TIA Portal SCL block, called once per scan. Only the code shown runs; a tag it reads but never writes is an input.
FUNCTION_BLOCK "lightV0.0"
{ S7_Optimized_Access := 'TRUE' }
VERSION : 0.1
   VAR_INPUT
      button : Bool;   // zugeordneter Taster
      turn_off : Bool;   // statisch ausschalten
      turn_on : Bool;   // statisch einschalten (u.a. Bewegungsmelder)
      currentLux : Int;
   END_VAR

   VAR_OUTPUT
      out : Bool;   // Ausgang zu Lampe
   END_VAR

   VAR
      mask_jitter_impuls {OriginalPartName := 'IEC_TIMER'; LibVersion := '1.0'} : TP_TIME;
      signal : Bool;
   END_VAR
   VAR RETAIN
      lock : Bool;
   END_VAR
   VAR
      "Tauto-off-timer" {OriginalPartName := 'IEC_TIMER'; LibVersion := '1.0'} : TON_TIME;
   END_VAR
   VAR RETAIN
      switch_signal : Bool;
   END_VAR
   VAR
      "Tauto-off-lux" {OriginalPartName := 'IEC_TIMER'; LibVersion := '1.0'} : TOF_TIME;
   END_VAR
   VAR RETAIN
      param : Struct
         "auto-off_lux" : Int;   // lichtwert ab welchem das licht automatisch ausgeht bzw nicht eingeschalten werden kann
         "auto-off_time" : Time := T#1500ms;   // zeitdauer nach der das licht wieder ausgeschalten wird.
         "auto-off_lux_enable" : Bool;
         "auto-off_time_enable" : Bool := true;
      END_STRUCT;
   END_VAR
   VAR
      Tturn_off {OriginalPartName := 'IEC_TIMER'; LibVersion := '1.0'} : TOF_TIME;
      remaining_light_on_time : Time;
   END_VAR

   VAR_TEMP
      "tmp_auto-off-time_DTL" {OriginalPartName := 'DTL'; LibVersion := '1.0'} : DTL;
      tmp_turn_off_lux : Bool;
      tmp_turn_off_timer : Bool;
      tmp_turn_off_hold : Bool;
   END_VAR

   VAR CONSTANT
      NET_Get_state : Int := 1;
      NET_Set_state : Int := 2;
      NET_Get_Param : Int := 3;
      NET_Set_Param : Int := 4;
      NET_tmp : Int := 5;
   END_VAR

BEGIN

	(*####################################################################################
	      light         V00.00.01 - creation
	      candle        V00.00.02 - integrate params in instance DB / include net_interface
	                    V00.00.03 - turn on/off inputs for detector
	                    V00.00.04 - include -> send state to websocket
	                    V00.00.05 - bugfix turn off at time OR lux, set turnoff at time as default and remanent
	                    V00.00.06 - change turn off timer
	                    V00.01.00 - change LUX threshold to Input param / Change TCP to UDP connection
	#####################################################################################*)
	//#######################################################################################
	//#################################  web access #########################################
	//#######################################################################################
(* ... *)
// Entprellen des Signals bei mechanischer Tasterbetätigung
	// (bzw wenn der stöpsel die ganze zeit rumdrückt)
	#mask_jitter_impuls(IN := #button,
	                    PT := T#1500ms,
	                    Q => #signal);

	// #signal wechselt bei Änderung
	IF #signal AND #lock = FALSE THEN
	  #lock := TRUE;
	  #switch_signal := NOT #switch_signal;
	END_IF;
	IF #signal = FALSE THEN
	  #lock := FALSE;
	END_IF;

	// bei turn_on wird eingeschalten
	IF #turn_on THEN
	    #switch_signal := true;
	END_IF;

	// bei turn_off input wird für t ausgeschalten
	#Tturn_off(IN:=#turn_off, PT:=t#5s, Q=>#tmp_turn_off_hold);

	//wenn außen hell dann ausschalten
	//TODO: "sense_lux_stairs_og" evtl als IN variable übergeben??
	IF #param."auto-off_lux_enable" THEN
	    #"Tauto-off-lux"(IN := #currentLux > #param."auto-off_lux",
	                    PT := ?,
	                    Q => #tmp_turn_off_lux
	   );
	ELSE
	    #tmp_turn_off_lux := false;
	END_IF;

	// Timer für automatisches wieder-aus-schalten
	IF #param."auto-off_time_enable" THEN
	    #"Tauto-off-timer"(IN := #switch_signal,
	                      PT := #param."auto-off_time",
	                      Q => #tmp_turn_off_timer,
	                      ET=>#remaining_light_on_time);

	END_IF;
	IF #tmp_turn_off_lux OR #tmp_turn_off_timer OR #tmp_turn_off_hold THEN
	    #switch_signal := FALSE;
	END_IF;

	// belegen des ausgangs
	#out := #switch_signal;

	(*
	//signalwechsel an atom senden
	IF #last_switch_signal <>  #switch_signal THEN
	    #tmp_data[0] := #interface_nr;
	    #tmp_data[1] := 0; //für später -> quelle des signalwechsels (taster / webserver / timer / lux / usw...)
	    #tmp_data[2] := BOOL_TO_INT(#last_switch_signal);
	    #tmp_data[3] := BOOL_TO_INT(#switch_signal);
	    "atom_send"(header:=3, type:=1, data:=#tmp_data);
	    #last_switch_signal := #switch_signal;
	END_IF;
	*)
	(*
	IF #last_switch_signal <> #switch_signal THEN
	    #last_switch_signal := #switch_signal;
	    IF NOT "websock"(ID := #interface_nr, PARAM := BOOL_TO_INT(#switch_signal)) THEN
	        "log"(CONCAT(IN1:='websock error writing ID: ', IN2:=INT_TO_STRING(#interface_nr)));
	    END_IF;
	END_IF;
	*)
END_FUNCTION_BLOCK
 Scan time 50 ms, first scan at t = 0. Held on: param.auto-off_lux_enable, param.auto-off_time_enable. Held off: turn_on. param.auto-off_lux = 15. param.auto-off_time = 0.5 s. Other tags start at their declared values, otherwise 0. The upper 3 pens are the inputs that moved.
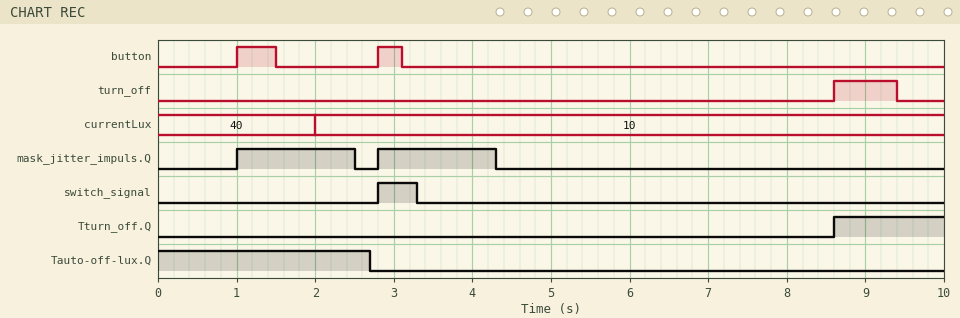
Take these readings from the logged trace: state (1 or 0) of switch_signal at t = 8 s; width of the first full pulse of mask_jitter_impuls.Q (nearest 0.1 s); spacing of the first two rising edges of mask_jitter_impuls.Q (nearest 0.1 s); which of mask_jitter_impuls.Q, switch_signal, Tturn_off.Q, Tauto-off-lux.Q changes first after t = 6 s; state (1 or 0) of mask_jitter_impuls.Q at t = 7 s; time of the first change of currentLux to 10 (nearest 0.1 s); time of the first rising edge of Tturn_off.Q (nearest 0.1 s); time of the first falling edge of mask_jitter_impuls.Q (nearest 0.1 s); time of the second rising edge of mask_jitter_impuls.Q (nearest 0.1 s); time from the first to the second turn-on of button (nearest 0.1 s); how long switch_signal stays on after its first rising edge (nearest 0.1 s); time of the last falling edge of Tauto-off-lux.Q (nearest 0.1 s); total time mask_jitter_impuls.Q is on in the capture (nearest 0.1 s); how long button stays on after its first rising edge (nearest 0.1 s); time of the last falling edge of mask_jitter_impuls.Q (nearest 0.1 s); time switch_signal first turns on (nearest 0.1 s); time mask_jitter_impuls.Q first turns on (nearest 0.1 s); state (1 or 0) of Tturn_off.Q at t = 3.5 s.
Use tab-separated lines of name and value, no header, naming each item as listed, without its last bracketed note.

state (1 or 0) of switch_signal at t = 8 s	0
width of the first full pulse of mask_jitter_impuls.Q	1.5 s
spacing of the first two rising edges of mask_jitter_impuls.Q	1.8 s
which of mask_jitter_impuls.Q, switch_signal, Tturn_off.Q, Tauto-off-lux.Q changes first after t = 6 s	Tturn_off.Q
state (1 or 0) of mask_jitter_impuls.Q at t = 7 s	0
time of the first change of currentLux to 10	2.0 s
time of the first rising edge of Tturn_off.Q	8.6 s
time of the first falling edge of mask_jitter_impuls.Q	2.5 s
time of the second rising edge of mask_jitter_impuls.Q	2.8 s
time from the first to the second turn-on of button	1.8 s
how long switch_signal stays on after its first rising edge	0.5 s
time of the last falling edge of Tauto-off-lux.Q	2.7 s
total time mask_jitter_impuls.Q is on in the capture	3.0 s
how long button stays on after its first rising edge	0.5 s
time of the last falling edge of mask_jitter_impuls.Q	4.3 s
time switch_signal first turns on	2.8 s
time mask_jitter_impuls.Q first turns on	1.0 s
state (1 or 0) of Tturn_off.Q at t = 3.5 s	0
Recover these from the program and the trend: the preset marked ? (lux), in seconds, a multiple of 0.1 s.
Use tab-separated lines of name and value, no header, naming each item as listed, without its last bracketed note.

the preset marked ? (lux), in seconds, a multiple of 0.1 s	0.7 s
